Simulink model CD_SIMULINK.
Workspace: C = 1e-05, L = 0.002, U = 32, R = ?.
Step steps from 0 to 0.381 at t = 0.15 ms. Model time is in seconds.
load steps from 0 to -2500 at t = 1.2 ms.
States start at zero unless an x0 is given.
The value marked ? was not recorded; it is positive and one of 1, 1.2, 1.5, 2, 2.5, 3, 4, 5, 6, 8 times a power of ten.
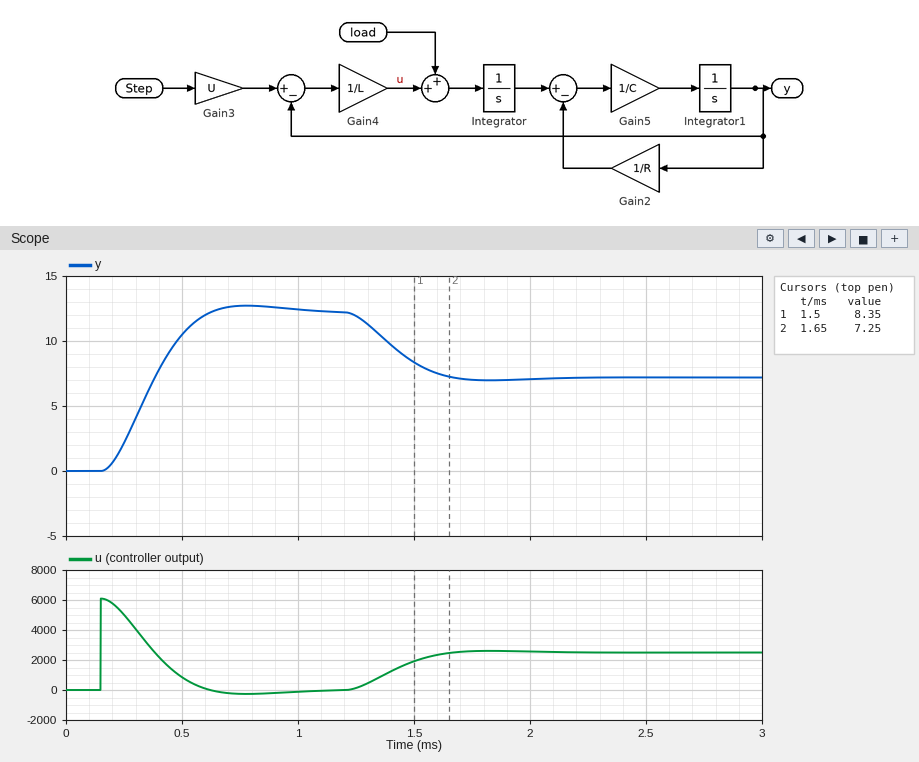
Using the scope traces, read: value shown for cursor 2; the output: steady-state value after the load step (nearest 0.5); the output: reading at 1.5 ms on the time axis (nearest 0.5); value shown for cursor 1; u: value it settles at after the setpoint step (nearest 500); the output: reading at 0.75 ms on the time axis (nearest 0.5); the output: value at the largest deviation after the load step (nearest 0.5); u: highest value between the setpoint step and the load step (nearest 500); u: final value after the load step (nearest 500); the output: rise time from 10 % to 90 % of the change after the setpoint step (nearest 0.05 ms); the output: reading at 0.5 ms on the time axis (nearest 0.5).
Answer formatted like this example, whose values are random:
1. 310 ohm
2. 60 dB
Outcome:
1. 7.25
2. 7.0
3. 8.5
4. 8.35
5. 0
6. 12.5
7. 7.0
8. 6000
9. 2500
10. 0.30 ms
11. 10.5
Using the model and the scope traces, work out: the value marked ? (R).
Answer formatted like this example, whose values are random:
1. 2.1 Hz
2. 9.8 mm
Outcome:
1. 10
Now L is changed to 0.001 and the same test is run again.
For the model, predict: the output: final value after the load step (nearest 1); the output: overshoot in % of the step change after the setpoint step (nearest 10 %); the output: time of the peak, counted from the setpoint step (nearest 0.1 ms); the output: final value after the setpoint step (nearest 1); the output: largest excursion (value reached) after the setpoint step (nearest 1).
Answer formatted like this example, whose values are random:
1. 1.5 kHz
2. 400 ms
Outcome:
1. 10
2. 20 %
3. 0.4 ms
4. 12
5. 14
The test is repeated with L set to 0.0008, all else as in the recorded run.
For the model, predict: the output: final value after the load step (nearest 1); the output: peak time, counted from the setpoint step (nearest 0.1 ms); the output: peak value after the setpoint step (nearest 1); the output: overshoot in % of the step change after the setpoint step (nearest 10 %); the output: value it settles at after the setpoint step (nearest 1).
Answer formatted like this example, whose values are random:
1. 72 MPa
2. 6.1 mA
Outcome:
1. 10
2. 0.3 ms
3. 15
4. 20 %
5. 12
